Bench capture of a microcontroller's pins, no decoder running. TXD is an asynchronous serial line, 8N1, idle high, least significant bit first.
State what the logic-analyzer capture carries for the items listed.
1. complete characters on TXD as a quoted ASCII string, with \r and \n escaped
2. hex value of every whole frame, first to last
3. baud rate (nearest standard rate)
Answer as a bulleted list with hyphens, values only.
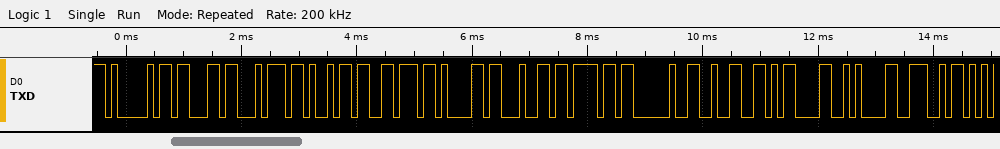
- "Activado 2\r\nN"
- 0x41 0x63 0x74 0x69 0x76 0x61 0x64 0x6F 0x20 0x32 0x0D 0x0A 0x4E
- 9600 baud
